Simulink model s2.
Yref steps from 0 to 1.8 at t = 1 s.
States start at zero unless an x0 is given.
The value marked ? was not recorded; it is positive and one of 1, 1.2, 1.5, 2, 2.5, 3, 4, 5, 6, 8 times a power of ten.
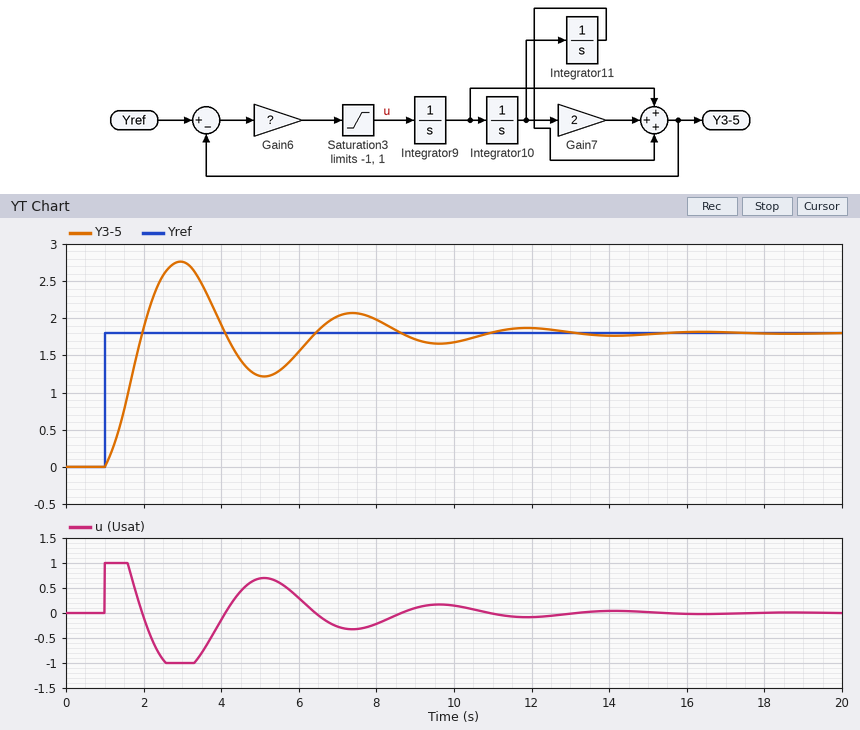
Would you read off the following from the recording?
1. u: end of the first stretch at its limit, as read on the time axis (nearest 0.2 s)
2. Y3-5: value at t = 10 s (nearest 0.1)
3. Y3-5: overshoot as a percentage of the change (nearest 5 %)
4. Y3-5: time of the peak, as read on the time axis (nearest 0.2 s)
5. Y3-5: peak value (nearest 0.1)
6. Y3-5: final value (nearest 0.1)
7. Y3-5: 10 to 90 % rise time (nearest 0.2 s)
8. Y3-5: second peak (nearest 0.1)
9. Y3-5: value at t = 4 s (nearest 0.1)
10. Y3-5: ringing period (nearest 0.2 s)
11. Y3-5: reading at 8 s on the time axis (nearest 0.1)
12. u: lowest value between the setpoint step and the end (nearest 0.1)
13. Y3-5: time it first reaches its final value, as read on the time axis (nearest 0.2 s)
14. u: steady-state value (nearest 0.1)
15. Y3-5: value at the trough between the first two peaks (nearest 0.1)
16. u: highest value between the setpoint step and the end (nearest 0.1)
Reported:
1.6 s
1.7
55 %
3.0 s
2.8
1.8
0.8 s
2.1
1.9
4.4 s
2.0
-1.0
2.0 s
0.0
1.2
1.0
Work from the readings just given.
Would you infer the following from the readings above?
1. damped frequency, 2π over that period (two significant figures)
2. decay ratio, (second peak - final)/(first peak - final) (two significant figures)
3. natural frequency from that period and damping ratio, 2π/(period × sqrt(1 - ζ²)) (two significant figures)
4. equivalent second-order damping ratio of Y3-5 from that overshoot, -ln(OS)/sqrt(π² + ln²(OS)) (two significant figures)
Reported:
1.4 rad/s
0.30
1.5 rad/s
0.19
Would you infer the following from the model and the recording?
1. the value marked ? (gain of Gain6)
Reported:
1.2
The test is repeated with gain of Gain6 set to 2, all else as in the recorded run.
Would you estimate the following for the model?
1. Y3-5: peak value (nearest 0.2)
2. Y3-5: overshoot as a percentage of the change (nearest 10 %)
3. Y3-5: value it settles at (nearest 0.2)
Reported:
2.6
40 %
1.8
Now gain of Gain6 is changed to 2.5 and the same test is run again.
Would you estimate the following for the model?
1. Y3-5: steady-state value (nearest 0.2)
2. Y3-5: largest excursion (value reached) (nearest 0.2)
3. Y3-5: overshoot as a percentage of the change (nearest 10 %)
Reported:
1.8
2.6
40 %
